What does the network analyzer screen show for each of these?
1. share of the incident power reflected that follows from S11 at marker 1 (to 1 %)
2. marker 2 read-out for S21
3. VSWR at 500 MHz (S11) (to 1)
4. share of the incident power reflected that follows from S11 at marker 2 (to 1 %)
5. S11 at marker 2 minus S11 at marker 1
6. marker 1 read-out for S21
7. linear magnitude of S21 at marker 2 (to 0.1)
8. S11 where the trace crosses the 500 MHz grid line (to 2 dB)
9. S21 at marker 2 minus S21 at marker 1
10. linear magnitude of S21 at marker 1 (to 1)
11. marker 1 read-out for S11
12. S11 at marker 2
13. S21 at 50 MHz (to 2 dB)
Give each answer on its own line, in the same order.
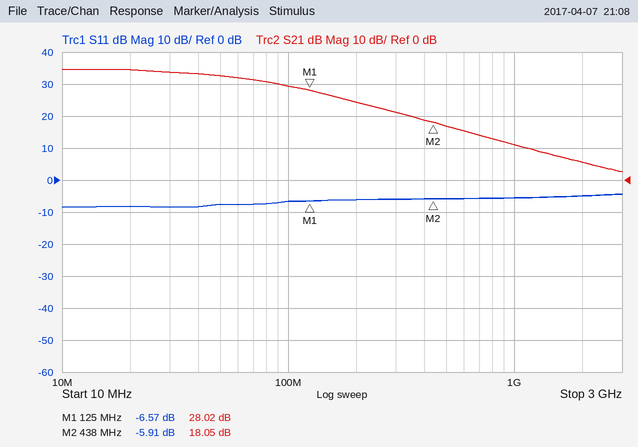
22 %
18.05 dB
3
26 %
0.66 dB
28.02 dB
8.0
-6 dB
-9.97 dB
25
-6.57 dB
-5.91 dB
32 dB
